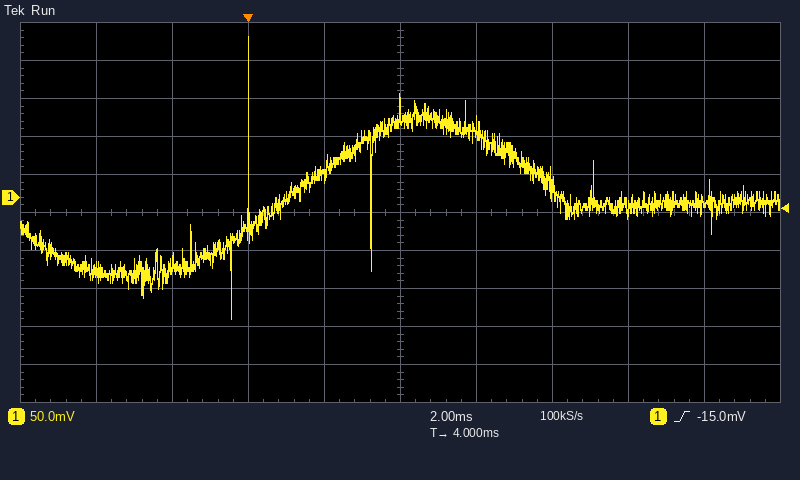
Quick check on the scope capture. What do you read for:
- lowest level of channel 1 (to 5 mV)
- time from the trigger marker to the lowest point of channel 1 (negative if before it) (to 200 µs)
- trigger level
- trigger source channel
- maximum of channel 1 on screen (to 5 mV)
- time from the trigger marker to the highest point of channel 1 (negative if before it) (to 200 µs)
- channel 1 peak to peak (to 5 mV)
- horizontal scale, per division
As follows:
-160 mV
-400 µs
-15.0 mV
channel 1
210 mV
0.0 ms
370 mV
2 ms
